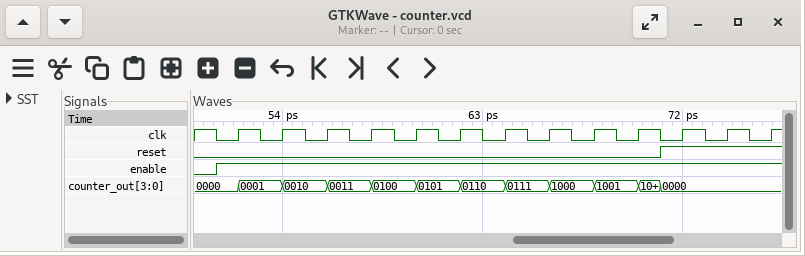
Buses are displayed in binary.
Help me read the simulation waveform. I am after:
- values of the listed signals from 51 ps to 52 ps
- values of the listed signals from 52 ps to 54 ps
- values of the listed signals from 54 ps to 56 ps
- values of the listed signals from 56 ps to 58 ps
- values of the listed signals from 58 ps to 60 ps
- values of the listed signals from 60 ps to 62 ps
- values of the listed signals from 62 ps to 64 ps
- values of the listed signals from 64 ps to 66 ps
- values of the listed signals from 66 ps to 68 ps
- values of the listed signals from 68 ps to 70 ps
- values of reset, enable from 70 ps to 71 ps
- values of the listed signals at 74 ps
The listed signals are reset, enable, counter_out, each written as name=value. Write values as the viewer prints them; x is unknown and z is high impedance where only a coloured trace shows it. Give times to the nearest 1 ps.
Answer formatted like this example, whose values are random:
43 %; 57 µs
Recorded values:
reset=0, enable=1, counter_out=0000; reset=0, enable=1, counter_out=0001; reset=0, enable=1, counter_out=0010; reset=0, enable=1, counter_out=0011; reset=0, enable=1, counter_out=0100; reset=0, enable=1, counter_out=0101; reset=0, enable=1, counter_out=0110; reset=0, enable=1, counter_out=0111; reset=0, enable=1, counter_out=1000; reset=0, enable=1, counter_out=1001; reset=0, enable=1; reset=1, enable=1, counter_out=0000
